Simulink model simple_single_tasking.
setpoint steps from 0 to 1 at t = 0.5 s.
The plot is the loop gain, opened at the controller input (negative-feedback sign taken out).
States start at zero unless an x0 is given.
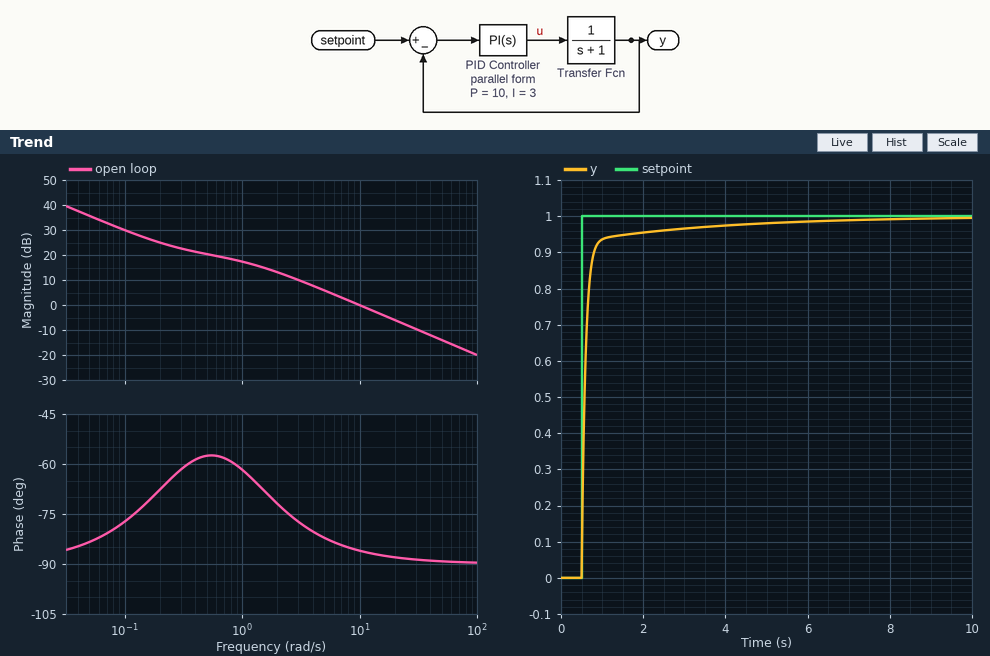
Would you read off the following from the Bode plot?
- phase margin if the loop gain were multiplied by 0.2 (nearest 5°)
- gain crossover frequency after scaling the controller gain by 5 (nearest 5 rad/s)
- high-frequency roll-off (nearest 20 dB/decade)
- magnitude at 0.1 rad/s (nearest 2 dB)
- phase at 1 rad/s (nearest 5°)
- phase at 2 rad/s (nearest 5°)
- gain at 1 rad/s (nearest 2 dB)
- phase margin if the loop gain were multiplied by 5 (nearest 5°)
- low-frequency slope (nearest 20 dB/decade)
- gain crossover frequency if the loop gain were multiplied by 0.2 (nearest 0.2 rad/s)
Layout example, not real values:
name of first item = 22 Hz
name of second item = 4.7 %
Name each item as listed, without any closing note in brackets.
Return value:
phase margin if the loop gain were multiplied by 0.2 = 110°
gain crossover frequency after scaling the controller gain by 5 = 50 rad/s
high-frequency roll-off = -20 dB/decade
magnitude at 0.1 rad/s = 30 dB
phase at 1 rad/s = -60°
phase at 2 rad/s = -70°
gain at 1 rad/s = 18 dB
phase margin if the loop gain were multiplied by 5 = 90°
low-frequency slope = -20 dB/decade
gain crossover frequency if the loop gain were multiplied by 0.2 = 1.8 rad/s
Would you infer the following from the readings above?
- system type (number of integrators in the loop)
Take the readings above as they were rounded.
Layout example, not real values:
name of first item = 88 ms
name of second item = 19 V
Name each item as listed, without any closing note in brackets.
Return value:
system type = 1
